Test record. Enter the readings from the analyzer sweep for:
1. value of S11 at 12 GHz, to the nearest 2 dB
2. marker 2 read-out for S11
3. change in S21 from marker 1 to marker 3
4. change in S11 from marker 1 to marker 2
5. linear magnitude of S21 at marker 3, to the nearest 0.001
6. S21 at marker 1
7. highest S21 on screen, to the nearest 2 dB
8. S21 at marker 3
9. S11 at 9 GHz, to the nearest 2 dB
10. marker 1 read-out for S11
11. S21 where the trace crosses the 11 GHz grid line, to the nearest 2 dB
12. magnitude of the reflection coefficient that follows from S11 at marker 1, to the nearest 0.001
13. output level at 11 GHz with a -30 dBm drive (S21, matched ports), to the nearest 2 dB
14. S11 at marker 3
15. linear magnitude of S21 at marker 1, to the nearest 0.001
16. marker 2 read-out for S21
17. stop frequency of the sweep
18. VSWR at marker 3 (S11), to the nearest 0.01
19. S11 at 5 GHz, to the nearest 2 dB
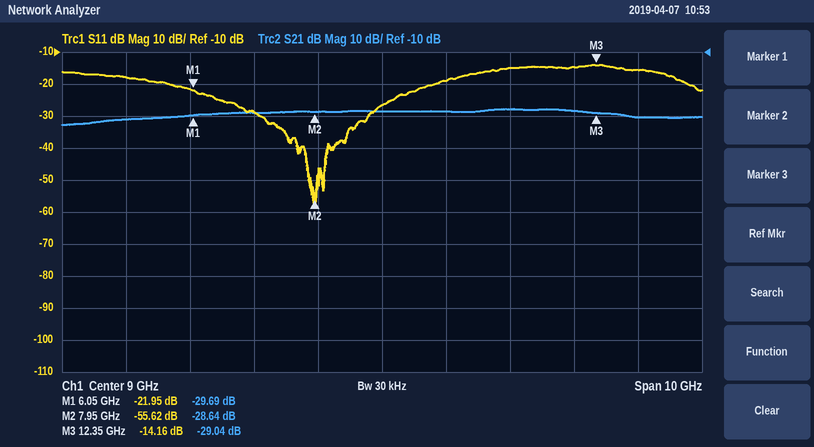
-14 dB
-55.62 dB
0.65 dB
-33.67 dB
0.035
-29.69 dB
-28 dB
-29.04 dB
-26 dB
-21.95 dB
-28 dB
0.080
-58 dBm
-14.16 dB
0.033
-28.64 dB
14 GHz
1.49
-18 dB
